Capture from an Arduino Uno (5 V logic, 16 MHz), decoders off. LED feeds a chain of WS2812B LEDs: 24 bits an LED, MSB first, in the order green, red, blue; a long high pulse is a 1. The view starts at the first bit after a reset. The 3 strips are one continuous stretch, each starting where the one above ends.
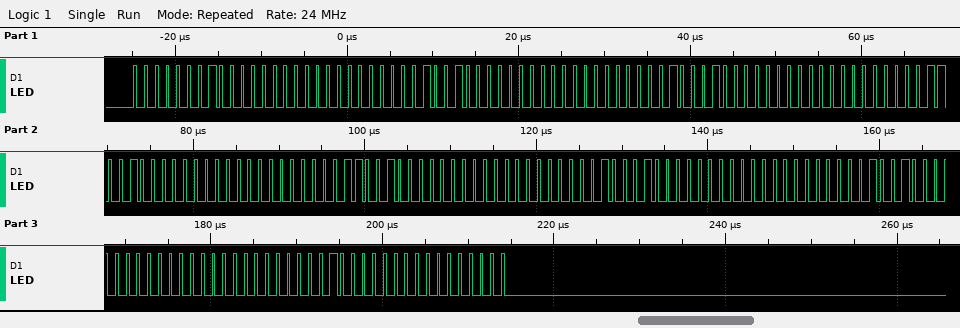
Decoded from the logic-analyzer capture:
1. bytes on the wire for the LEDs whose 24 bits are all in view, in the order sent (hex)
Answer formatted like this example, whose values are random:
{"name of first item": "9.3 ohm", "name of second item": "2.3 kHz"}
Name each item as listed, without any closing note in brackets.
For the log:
{"bytes on the wire for the LEDs whose 24 bits are all in view, in the order sent": "01 00 00 12 00 00 22 00 00 32 00 00 32 00 00 22 00 00 12 00 00 01 00 00"}
